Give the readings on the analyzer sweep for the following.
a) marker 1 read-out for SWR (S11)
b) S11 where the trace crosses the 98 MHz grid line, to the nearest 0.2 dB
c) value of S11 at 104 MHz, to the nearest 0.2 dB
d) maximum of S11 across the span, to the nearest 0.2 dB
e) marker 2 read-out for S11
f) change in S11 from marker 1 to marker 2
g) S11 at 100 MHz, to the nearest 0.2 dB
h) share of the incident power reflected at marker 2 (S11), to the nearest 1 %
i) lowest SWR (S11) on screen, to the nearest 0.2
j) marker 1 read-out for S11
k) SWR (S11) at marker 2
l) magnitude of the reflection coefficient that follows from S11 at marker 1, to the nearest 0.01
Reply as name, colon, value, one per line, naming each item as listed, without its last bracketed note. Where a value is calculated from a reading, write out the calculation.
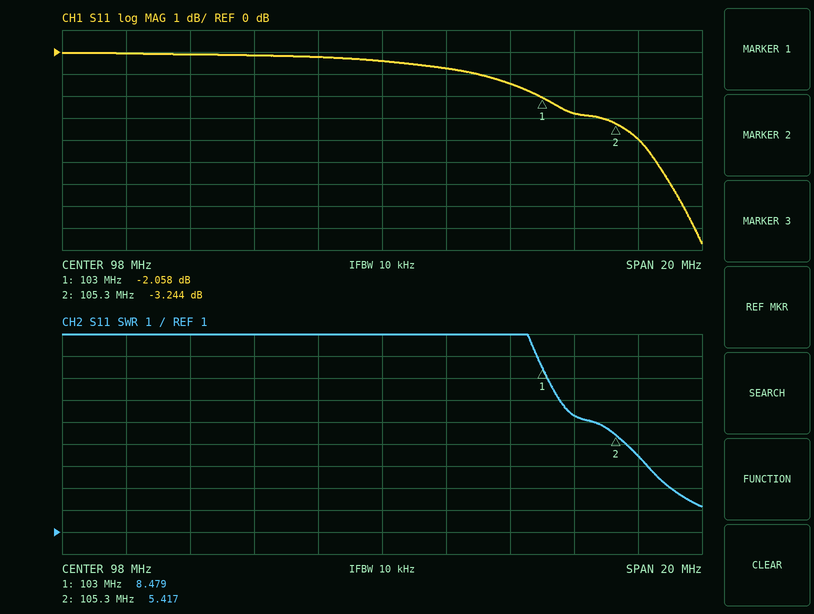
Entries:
marker 1 read-out for SWR: 8.479
S11 where the trace crosses the 98 MHz grid line, to the nearest 0.2 dB: -0.4 dB
value of S11 at 104 MHz, to the nearest 0.2 dB: -2.8 dB
maximum of S11 across the span, to the nearest 0.2 dB: 0.0 dB
marker 2 read-out for S11: -3.244 dB
change in S11 from marker 1 to marker 2: -3.244 − (-2.058) = -1.186 dB
S11 at 100 MHz, to the nearest 0.2 dB: -0.8 dB
share of the incident power reflected at marker 2 (S11), to the nearest 1 %: 10^(-3.244/10) ≈ 47 %
lowest SWR (S11) on screen, to the nearest 0.2: 2.2
marker 1 read-out for S11: -2.058 dB
SWR (S11) at marker 2: 5.417
magnitude of the reflection coefficient that follows from S11 at marker 1, to the nearest 0.01: 10^(-2.058/20) ≈ 0.79
